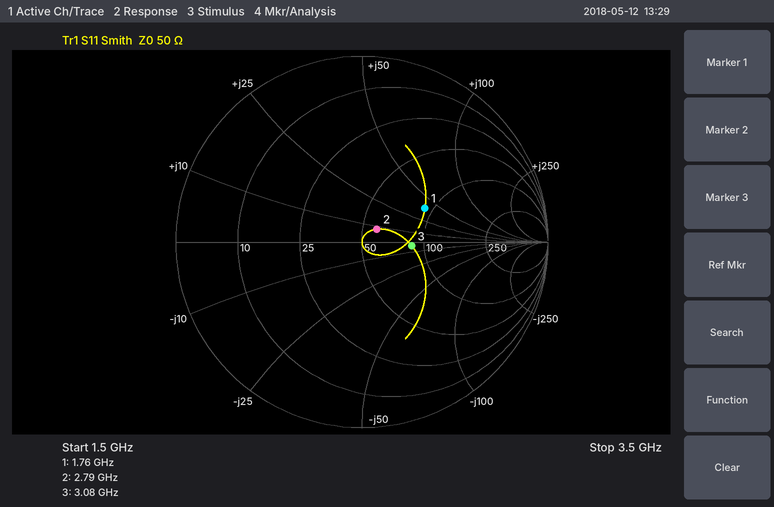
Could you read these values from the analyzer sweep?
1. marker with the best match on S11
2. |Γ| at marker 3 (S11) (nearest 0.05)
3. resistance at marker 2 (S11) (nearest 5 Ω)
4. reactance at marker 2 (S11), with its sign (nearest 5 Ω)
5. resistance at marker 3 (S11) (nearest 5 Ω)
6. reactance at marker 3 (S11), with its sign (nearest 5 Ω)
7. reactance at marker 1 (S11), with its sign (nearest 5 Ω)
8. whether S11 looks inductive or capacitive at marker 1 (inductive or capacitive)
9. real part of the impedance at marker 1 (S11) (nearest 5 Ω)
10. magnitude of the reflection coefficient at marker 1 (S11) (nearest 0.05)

marker 2
0.25
60 Ω
+10 Ω
85 Ω
-5 Ω
+40 Ω
inductive
90 Ω
0.40
